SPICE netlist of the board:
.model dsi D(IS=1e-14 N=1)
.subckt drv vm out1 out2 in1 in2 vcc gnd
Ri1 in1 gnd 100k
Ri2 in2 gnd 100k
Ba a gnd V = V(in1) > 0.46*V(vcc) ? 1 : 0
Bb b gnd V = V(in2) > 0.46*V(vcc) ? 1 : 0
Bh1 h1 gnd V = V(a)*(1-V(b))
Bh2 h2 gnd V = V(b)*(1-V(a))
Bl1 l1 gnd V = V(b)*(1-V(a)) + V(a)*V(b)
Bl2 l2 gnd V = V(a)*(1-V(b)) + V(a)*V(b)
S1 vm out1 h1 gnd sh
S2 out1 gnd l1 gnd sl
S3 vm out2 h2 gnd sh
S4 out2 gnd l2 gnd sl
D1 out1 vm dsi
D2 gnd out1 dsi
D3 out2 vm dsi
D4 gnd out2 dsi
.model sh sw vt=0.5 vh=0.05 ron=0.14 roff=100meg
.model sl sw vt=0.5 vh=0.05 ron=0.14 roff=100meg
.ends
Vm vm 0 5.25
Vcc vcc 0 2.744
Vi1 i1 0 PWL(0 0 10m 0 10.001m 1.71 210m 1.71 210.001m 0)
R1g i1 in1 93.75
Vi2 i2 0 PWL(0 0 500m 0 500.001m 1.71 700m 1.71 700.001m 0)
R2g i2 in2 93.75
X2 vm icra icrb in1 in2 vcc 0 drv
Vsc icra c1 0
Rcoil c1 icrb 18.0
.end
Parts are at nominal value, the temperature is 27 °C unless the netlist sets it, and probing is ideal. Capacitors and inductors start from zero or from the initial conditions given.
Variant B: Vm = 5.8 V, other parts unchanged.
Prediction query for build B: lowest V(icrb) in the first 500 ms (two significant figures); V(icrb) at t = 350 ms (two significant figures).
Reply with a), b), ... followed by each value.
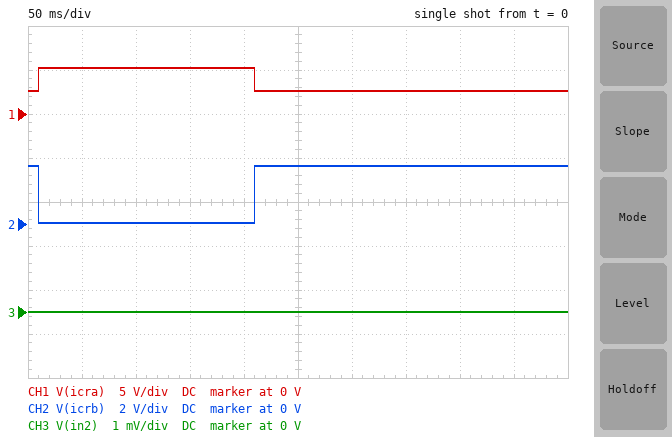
a) 44 mV
b) 2.9 V
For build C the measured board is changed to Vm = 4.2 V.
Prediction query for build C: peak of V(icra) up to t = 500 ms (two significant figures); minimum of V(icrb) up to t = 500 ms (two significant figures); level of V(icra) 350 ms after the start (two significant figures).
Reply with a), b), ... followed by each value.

a) 4.2 V
b) 32 mV
c) 2.1 V
